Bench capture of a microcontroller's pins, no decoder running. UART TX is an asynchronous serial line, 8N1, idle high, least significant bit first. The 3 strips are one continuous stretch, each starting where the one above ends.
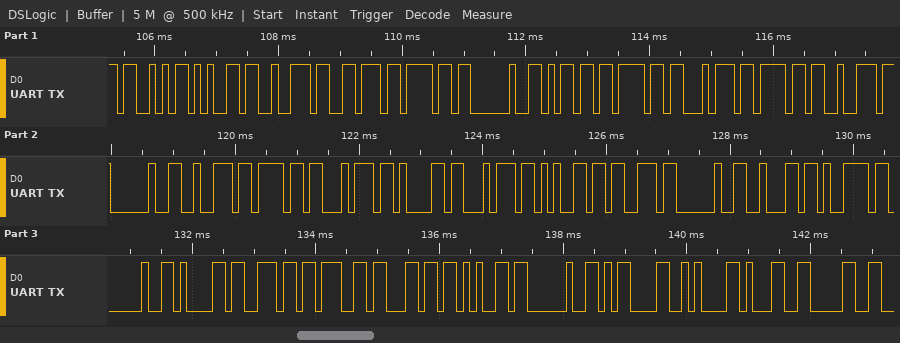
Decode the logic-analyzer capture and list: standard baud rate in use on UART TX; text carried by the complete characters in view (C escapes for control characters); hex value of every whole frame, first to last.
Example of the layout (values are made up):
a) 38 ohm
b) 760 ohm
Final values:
a) 9600 baud
b) "Servo motor rotates by angle \r\n10"
c) 53 65 72 76 6F 20 6D 6F 74 6F 72 20 72 6F 74 61 74 65 73 20 62 79 20 61 6E 67 6C 65 20 0D 0A 31 30
